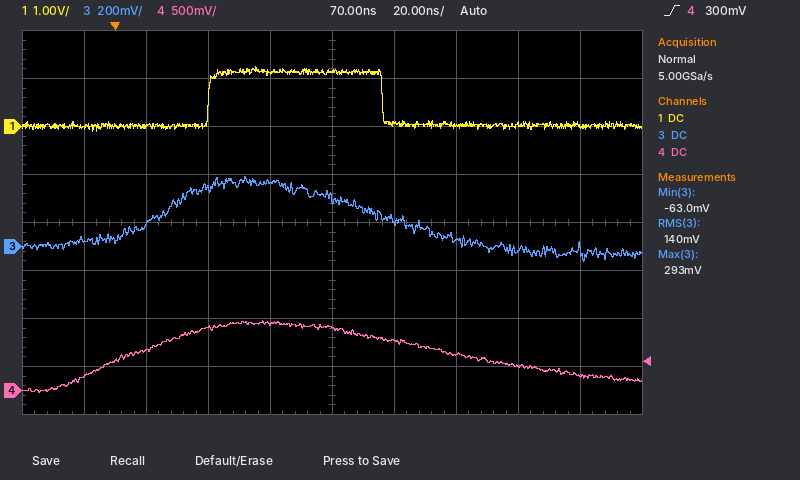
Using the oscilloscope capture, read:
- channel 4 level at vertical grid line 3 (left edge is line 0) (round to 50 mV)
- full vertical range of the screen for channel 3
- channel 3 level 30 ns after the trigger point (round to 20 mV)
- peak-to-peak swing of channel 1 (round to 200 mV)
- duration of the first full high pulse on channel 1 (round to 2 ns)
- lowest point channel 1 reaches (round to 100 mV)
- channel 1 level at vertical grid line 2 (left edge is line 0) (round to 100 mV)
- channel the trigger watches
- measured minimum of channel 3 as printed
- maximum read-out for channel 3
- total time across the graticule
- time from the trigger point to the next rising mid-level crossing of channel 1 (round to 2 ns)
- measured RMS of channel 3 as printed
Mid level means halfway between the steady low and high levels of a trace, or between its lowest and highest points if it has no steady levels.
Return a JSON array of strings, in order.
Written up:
["650 mV", "1.6 V", "240 mV", "1.4 V", "56 ns", "-100 mV", "0.0 V", "channel 4", "-63.0 mV", "293 mV", "200 ns", "30 ns", "140 mV"]
